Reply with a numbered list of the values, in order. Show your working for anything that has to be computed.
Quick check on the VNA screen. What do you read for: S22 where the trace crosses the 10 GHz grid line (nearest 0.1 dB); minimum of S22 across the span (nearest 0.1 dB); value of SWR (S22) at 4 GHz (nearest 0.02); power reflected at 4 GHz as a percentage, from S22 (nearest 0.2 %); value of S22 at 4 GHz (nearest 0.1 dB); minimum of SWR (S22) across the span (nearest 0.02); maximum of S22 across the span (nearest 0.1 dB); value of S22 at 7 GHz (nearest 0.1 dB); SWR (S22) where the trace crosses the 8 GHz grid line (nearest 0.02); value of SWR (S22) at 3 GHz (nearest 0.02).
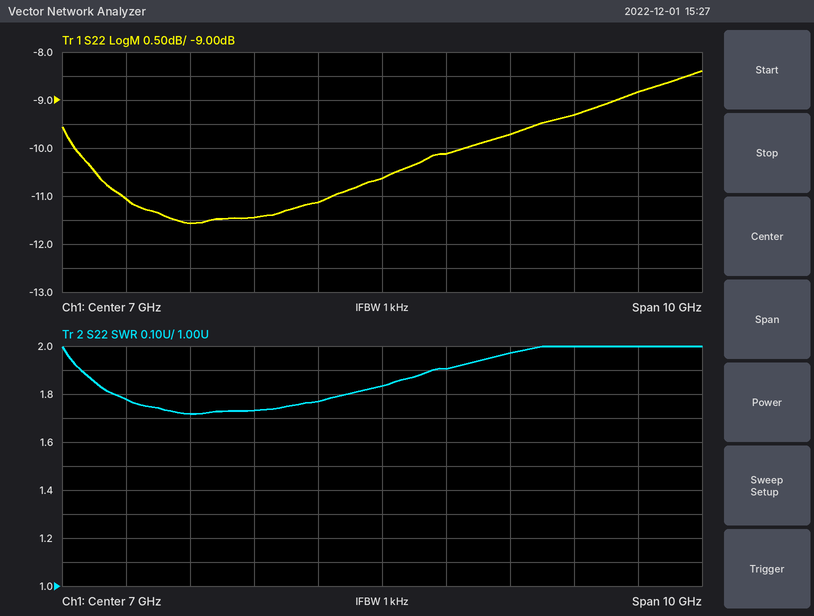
1. -9.3 dB
2. -11.6 dB
3. 1.72
4. 10^(-11.6/10) ≈ 6.92 %, so 7.0 % to the nearest 0.2 %
5. -11.6 dB
6. 1.72
7. -8.4 dB
8. -10.6 dB
9. 1.90
10. 1.78
